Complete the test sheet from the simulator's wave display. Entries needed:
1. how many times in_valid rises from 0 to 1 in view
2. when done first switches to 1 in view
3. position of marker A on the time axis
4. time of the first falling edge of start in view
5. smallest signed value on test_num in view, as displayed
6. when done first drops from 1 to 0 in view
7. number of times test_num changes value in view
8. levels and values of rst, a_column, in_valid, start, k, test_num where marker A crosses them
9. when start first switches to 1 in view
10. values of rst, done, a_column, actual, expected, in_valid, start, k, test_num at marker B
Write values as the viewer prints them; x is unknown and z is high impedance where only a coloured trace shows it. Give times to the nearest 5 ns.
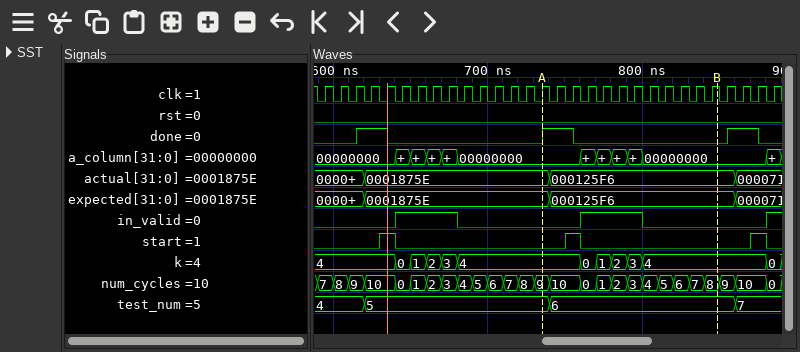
3
615 ns
735 ns
640 ns
4
635 ns
3
rst=0, a_column=00000000, in_valid=0, start=0, k=4, test_num=5
630 ns
rst=0, done=0, a_column=00000000, actual=000125F6, expected=000125F6, in_valid=0, start=0, k=4, test_num=6
